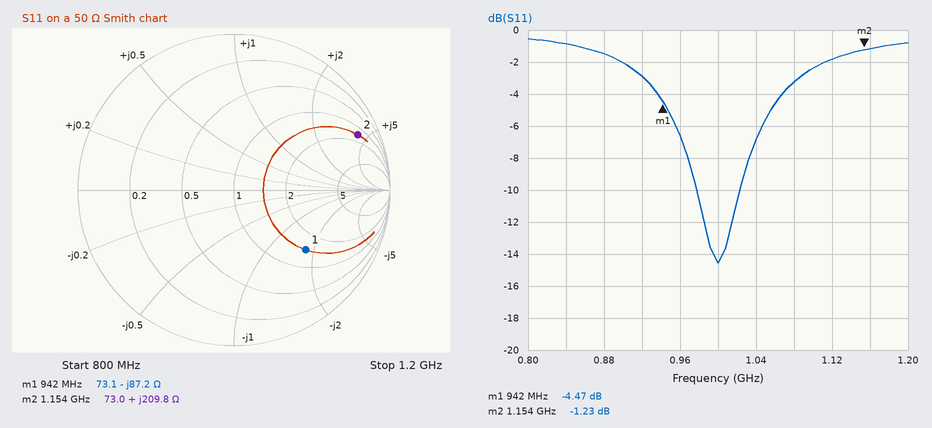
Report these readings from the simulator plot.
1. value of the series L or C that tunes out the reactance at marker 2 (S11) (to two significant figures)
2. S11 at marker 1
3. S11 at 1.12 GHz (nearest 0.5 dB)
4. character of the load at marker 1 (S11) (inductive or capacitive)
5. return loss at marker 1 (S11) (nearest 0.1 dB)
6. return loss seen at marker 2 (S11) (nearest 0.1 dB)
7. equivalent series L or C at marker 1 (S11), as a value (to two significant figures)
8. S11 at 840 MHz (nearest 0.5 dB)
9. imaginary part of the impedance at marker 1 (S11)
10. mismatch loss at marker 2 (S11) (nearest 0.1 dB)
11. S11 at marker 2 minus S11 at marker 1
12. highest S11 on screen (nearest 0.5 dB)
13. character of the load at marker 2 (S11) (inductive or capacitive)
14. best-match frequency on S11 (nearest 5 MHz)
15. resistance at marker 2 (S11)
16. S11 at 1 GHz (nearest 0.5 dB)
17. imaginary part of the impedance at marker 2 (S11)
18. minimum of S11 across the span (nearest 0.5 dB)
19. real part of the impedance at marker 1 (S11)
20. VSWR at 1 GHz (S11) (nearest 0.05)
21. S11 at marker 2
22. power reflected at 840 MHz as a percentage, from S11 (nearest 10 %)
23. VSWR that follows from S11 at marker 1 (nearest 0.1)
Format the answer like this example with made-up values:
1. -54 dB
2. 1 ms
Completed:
1. 660 fF
2. -4.47 dB
3. -2.0 dB
4. capacitive
5. 4.5 dB
6. 1.2 dB
7. 1.9 pF
8. -1.0 dB
9. -87.2 Ω
10. 6.1 dB
11. 3.24 dB
12. -0.5 dB
13. inductive
14. 1.000 GHz
15. 73.0 Ω
16. -14.5 dB
17. +209.8 Ω
18. -14.5 dB
19. 73.1 Ω
20. 1.45
21. -1.23 dB
22. 80 %
23. 4.0
